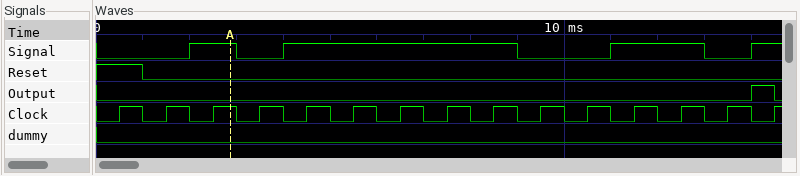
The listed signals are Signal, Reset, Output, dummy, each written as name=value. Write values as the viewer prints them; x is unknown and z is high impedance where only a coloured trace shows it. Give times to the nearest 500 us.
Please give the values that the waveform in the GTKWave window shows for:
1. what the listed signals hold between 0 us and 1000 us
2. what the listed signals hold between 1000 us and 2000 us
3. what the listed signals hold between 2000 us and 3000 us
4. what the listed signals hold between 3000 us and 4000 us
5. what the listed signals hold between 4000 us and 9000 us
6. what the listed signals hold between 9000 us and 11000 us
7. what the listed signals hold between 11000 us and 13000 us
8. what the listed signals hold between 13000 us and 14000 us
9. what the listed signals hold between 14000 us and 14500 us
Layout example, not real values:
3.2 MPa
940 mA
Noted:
Signal=0, Reset=1, Output=0, dummy=0
Signal=0, Reset=0, Output=0, dummy=0
Signal=1, Reset=0, Output=0, dummy=0
Signal=0, Reset=0, Output=0, dummy=0
Signal=1, Reset=0, Output=0, dummy=0
Signal=0, Reset=0, Output=0, dummy=0
Signal=1, Reset=0, Output=0, dummy=0
Signal=0, Reset=0, Output=0, dummy=0
Signal=1, Reset=0, Output=1, dummy=0
